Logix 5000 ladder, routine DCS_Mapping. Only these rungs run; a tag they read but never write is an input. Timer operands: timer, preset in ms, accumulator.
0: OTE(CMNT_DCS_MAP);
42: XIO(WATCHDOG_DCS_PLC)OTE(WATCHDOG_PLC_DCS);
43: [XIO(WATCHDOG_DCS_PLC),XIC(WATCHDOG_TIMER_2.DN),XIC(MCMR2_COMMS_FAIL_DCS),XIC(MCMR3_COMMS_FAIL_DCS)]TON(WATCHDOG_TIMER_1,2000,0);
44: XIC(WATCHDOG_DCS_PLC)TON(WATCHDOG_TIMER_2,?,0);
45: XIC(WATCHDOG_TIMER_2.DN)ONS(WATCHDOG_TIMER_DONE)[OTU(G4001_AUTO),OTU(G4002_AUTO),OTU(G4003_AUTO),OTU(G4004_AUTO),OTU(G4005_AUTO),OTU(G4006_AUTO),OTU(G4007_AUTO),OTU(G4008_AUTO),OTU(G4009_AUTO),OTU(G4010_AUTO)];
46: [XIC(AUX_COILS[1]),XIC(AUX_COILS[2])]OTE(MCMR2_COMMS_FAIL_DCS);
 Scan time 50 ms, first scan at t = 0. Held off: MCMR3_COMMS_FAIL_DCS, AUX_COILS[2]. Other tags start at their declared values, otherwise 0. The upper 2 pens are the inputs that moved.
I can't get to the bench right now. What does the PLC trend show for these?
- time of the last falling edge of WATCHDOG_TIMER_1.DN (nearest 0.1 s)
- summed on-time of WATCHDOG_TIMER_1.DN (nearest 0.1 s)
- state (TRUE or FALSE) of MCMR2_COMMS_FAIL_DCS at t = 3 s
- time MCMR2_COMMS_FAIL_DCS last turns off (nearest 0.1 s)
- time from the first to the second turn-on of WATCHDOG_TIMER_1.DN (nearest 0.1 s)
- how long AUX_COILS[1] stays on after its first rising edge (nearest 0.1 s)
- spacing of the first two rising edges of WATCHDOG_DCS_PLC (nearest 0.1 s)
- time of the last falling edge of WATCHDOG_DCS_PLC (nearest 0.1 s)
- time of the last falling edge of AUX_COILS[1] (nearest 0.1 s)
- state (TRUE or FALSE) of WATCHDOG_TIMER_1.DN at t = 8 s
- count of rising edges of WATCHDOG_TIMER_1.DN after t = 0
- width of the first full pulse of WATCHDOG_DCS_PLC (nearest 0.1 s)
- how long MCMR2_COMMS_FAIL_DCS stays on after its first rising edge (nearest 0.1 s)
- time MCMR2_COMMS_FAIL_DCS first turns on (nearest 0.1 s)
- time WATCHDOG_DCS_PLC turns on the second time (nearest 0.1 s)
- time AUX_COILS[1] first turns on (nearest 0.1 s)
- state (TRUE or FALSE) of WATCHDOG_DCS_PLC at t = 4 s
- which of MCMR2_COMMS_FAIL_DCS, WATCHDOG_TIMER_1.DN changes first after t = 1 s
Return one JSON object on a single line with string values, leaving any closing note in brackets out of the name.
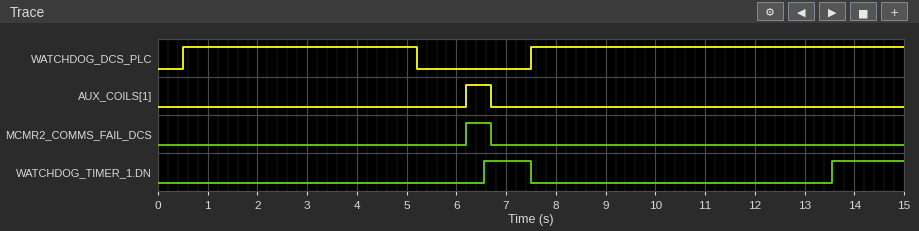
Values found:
{"time of the last falling edge of WATCHDOG_TIMER_1.DN": "7.5 s", "summed on-time of WATCHDOG_TIMER_1.DN": "2.4 s", "state (TRUE or FALSE) of MCMR2_COMMS_FAIL_DCS at t = 3 s": "FALSE", "time MCMR2_COMMS_FAIL_DCS last turns off": "6.7 s", "time from the first to the second turn-on of WATCHDOG_TIMER_1.DN": "7.0 s", "how long AUX_COILS[1] stays on after its first rising edge": "0.5 s", "spacing of the first two rising edges of WATCHDOG_DCS_PLC": "7.0 s", "time of the last falling edge of WATCHDOG_DCS_PLC": "5.2 s", "time of the last falling edge of AUX_COILS[1]": "6.7 s", "state (TRUE or FALSE) of WATCHDOG_TIMER_1.DN at t = 8 s": "FALSE", "count of rising edges of WATCHDOG_TIMER_1.DN after t = 0": "2", "width of the first full pulse of WATCHDOG_DCS_PLC": "4.7 s", "how long MCMR2_COMMS_FAIL_DCS stays on after its first rising edge": "0.5 s", "time MCMR2_COMMS_FAIL_DCS first turns on": "6.2 s", "time WATCHDOG_DCS_PLC turns on the second time": "7.5 s", "time AUX_COILS[1] first turns on": "6.2 s", "state (TRUE or FALSE) of WATCHDOG_DCS_PLC at t = 4 s": "TRUE", "which of MCMR2_COMMS_FAIL_DCS, WATCHDOG_TIMER_1.DN changes first after t = 1 s": "MCMR2_COMMS_FAIL_DCS"}
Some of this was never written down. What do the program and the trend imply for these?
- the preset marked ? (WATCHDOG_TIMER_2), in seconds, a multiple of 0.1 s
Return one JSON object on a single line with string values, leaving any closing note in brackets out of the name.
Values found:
{"the preset marked ? (WATCHDOG_TIMER_2), in seconds, a multiple of 0.1 s": "4.0 s"}
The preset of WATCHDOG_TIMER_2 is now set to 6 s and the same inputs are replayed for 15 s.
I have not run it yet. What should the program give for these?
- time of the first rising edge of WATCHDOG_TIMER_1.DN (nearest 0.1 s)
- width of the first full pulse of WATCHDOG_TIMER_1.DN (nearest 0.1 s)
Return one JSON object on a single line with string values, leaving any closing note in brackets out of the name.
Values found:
{"time of the first rising edge of WATCHDOG_TIMER_1.DN": "7.2 s", "width of the first full pulse of WATCHDOG_TIMER_1.DN": "0.3 s"}
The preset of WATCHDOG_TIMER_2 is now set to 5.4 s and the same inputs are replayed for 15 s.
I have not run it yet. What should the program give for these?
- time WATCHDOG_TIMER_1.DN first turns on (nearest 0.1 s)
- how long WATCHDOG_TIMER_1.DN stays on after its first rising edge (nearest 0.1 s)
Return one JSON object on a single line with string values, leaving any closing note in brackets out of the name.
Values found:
{"time WATCHDOG_TIMER_1.DN first turns on": "7.2 s", "how long WATCHDOG_TIMER_1.DN stays on after its first rising edge": "0.3 s"}
